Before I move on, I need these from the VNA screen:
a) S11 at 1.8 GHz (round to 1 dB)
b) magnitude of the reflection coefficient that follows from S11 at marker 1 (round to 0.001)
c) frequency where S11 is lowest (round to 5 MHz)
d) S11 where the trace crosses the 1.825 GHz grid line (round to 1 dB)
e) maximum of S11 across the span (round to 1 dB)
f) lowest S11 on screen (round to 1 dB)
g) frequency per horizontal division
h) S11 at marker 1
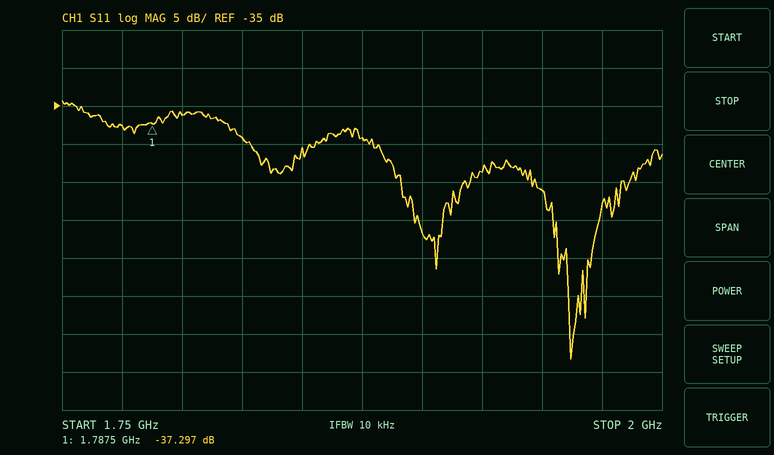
-36 dB
0.014
1.960 GHz
-39 dB
-34 dB
-68 dB
25 MHz
-37.297 dB
